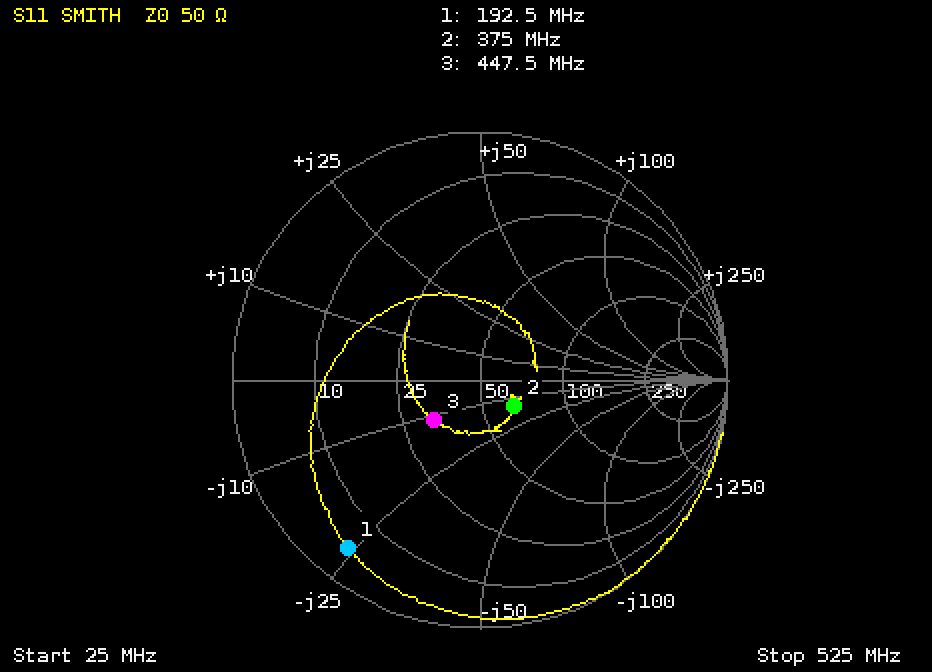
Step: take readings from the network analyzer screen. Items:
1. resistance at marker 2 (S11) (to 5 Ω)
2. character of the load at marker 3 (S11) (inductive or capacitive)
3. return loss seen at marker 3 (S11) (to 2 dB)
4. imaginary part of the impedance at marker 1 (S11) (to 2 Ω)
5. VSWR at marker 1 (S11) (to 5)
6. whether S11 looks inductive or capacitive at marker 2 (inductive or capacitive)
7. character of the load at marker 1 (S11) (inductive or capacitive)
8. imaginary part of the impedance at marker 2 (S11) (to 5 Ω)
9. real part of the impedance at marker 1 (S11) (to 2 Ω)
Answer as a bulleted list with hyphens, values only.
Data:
- 65 Ω
- capacitive
- 12 dB
- -24 Ω
- 15
- capacitive
- capacitive
- -15 Ω
- 4 Ω
